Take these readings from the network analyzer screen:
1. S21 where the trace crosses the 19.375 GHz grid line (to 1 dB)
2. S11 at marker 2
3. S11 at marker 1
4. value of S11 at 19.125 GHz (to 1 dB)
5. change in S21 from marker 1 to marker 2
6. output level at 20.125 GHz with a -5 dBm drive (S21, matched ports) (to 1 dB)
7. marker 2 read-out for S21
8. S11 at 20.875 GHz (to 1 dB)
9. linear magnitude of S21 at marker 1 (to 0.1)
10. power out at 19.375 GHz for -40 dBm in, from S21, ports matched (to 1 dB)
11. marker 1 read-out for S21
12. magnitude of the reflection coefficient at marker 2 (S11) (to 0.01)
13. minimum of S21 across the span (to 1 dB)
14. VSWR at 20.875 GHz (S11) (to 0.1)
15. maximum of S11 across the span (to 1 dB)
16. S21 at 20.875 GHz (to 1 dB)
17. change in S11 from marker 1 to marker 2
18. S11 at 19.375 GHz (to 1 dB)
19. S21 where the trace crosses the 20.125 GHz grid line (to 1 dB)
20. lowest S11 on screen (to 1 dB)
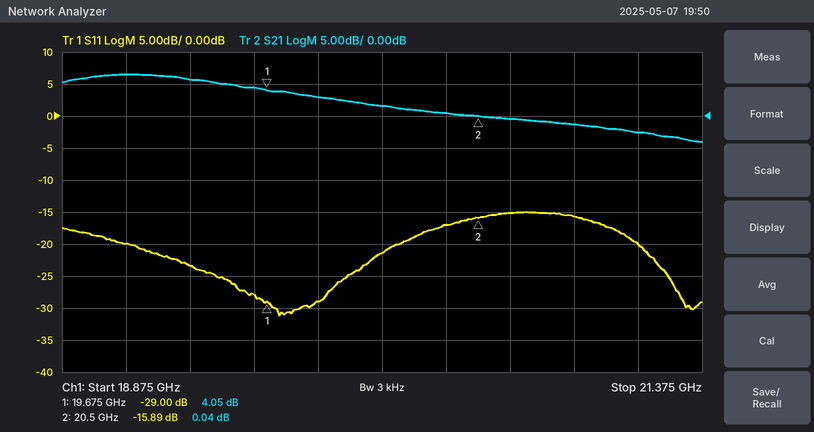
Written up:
6 dB
-15.89 dB
-29.00 dB
-20 dB
-4.01 dB
-3 dBm
0.04 dB
-16 dB
1.6
-34 dBm
4.05 dB
0.16
-4 dB
1.4
-15 dB
-1 dB
13.11 dB
-23 dB
2 dB
-31 dB
